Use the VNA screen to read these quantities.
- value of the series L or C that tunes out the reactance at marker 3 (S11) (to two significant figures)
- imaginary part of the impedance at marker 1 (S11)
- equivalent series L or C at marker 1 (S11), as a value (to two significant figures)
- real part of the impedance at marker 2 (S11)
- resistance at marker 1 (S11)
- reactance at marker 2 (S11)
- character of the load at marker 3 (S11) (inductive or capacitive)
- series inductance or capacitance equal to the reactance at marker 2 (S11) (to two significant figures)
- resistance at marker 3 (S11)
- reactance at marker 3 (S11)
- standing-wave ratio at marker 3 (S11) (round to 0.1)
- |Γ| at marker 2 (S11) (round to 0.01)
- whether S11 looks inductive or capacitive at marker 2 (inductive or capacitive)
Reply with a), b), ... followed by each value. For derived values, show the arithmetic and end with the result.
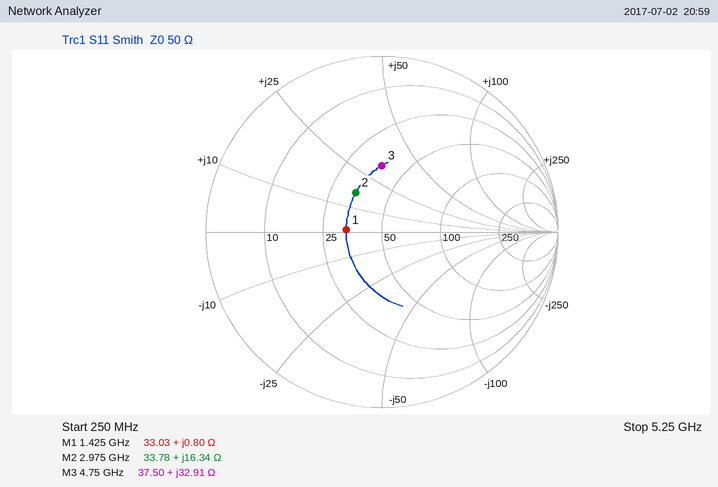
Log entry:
a) C = 1/(2π × 4.75 GHz × 32.91 Ω) ≈ 1.0 pF
b) +0.80 Ω
c) L = 0.8 Ω/(2π × 1.425 GHz) ≈ 89 pH
d) 33.78 Ω
e) 33.03 Ω
f) +16.34 Ω
g) inductive
h) L = 16.34 Ω/(2π × 2.975 GHz) ≈ 874 pH, so 870 pH to two significant figures
i) 37.50 Ω
j) +32.91 Ω
k) 2.2
l) 0.27
m) inductive
